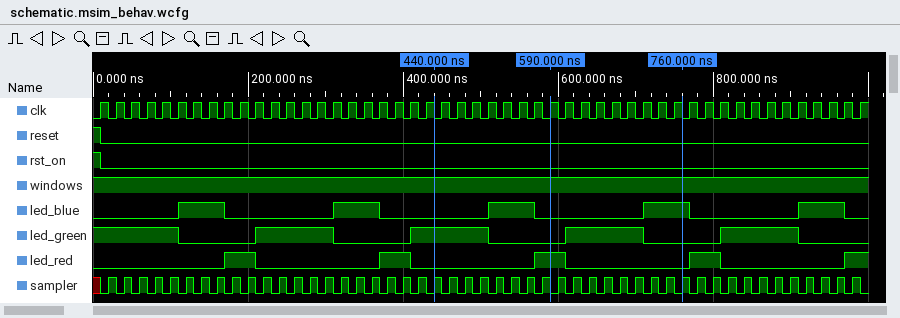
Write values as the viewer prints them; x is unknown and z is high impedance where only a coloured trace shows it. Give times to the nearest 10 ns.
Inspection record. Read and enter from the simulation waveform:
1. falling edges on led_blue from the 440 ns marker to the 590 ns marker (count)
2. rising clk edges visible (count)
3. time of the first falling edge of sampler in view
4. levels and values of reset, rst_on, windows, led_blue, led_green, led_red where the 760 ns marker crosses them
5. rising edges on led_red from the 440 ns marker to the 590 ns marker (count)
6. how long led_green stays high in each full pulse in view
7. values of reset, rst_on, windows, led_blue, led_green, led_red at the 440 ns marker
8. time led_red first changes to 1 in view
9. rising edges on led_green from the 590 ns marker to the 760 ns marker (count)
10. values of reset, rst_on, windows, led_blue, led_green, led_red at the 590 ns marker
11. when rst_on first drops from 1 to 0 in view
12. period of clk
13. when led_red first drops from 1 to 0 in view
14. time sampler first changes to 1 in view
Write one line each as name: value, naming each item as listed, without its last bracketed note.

falling edges on led_blue from the 440 ns marker to the 590 ns marker: 1
rising clk edges visible: 50
time of the first falling edge of sampler in view: 30 ns
levels and values of reset, rst_on, windows, led_blue, led_green, led_red where the 760 ns marker crosses them: reset=0, rst_on=0, windows=1, led_blue=1, led_green=0, led_red=0
rising edges on led_red from the 440 ns marker to the 590 ns marker: 1
how long led_green stays high in each full pulse in view: 100 ns, 100 ns, 100 ns, 100 ns
values of reset, rst_on, windows, led_blue, led_green, led_red at the 440 ns marker: reset=0, rst_on=0, windows=1, led_blue=0, led_green=1, led_red=0
time led_red first changes to 1 in view: 170 ns
rising edges on led_green from the 590 ns marker to the 760 ns marker: 1
values of reset, rst_on, windows, led_blue, led_green, led_red at the 590 ns marker: reset=0, rst_on=0, windows=1, led_blue=0, led_green=0, led_red=1
when rst_on first drops from 1 to 0 in view: 10 ns
period of clk: 20 ns
when led_red first drops from 1 to 0 in view: 210 ns
time sampler first changes to 1 in view: 20 ns
